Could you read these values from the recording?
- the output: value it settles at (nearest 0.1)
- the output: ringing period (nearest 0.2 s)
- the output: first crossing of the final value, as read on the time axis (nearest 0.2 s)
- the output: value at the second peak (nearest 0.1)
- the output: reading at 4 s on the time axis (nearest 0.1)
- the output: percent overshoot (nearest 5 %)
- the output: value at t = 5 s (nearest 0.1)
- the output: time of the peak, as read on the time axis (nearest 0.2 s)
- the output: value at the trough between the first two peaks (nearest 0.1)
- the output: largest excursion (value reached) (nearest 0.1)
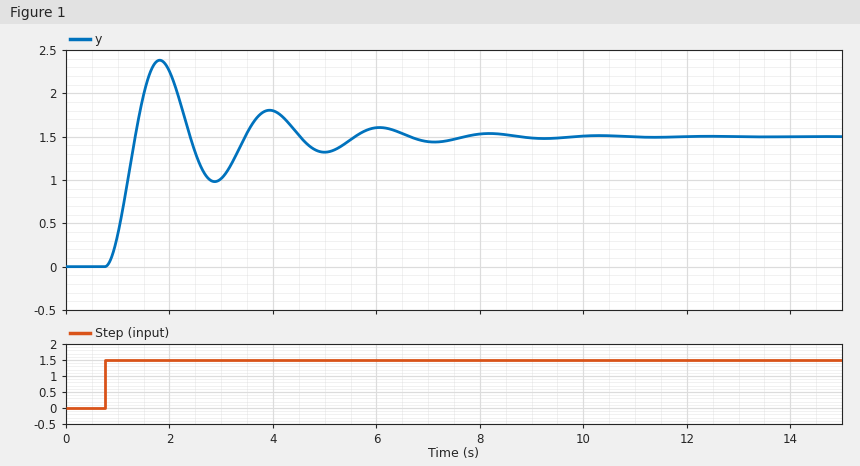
1.5
2.2 s
1.4 s
1.8
1.8
60 %
1.3
1.8 s
1.0
2.4
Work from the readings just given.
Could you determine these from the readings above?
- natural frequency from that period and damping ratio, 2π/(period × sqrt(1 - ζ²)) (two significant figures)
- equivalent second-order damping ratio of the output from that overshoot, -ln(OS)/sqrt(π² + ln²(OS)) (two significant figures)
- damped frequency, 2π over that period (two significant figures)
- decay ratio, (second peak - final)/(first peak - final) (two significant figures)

2.9 rad/s
0.16
2.9 rad/s
0.33
